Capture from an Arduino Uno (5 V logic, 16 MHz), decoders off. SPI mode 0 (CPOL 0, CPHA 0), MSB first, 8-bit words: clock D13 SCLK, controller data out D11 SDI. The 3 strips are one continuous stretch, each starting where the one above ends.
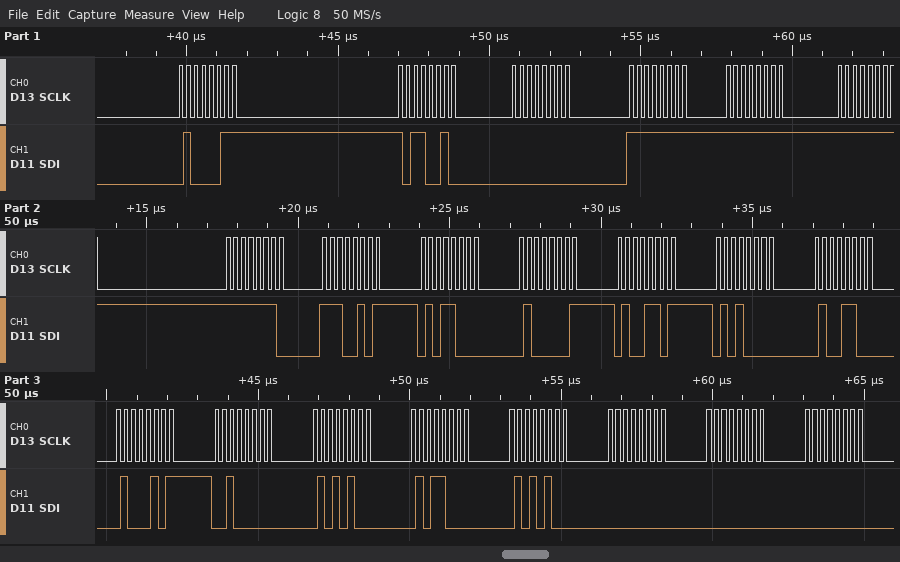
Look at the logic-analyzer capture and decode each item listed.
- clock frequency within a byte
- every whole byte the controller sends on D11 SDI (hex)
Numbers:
4 MHz
0x43 0xB2 0x00 0xFF 0xFF 0xFF 0xFE 0xE5 0x58 0x41 0x4D 0x50 0x4C 0x45 0x20 0x54 0x58 0x54 0x00 0x00 0x00
